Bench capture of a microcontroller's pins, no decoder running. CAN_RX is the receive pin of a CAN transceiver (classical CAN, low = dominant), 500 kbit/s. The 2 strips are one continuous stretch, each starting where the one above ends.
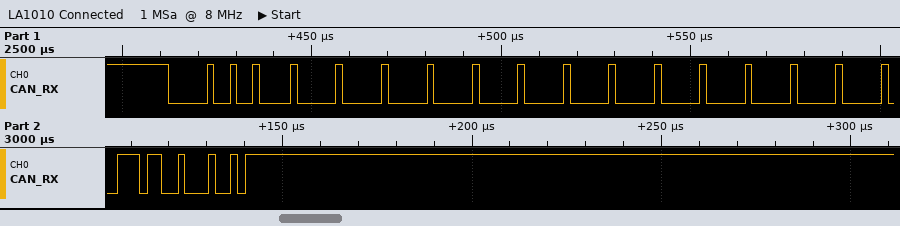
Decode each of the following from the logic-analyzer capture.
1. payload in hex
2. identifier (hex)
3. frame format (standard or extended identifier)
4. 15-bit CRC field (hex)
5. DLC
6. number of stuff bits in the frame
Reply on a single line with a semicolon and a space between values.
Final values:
00 00 00 00 00 00 00 00; 0x012; standard; 0x7644; 8; 14
